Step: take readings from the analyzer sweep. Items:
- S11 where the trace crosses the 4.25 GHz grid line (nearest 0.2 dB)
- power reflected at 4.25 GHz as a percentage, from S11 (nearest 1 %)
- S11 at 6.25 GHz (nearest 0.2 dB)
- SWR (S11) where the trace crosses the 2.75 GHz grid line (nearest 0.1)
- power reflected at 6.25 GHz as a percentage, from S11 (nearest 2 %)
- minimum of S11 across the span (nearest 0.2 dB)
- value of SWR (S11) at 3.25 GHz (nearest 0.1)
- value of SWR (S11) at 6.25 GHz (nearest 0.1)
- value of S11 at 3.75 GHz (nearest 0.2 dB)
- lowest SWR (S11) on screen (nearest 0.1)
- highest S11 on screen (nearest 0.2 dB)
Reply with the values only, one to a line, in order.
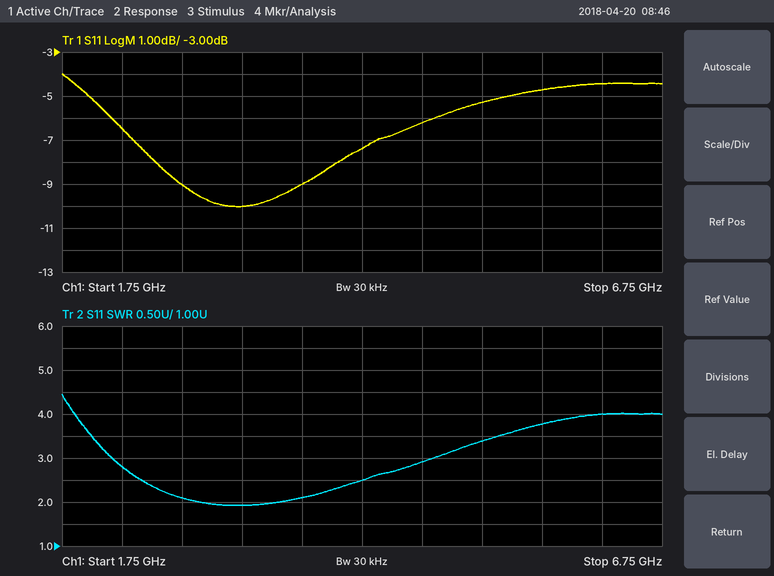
-7.4 dB
18 %
-4.4 dB
2.1
36 %
-10.0 dB
1.9
4.0
-9.0 dB
1.9
-4.0 dB
